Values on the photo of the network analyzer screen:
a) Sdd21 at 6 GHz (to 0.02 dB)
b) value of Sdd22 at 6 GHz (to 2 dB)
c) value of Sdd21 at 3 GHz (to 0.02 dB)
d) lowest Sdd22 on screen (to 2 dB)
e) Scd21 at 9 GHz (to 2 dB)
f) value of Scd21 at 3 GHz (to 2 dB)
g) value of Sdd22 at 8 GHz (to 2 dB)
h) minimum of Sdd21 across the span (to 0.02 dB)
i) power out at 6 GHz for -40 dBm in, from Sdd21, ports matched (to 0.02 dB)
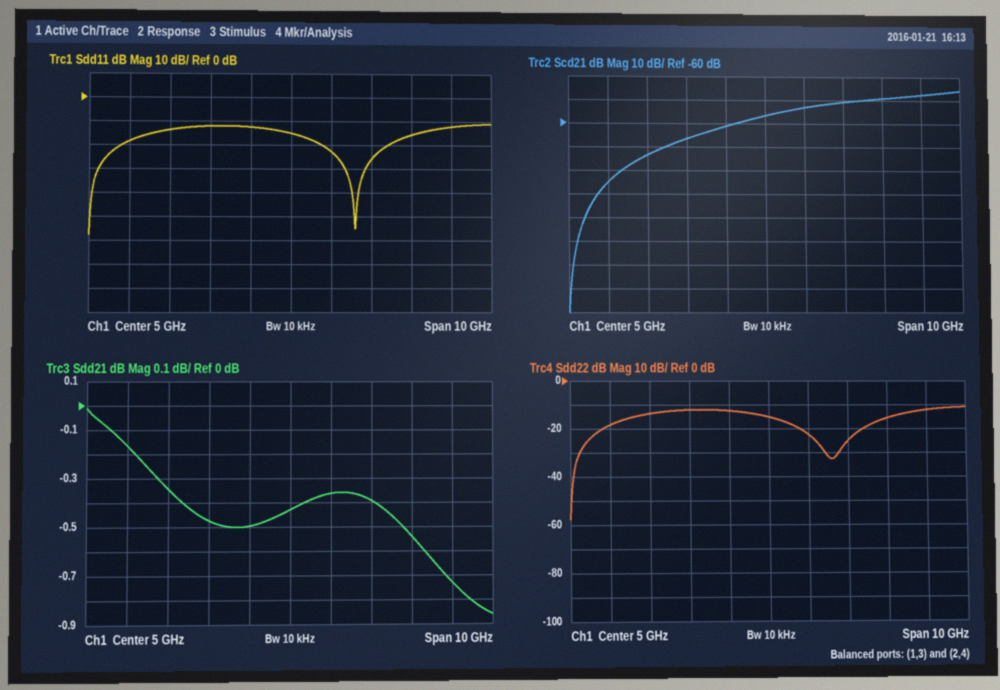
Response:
-0.36 dB
-22 dB
-0.48 dB
-58 dB
-48 dB
-66 dB
-16 dB
-0.86 dB
-40.36 dBm
